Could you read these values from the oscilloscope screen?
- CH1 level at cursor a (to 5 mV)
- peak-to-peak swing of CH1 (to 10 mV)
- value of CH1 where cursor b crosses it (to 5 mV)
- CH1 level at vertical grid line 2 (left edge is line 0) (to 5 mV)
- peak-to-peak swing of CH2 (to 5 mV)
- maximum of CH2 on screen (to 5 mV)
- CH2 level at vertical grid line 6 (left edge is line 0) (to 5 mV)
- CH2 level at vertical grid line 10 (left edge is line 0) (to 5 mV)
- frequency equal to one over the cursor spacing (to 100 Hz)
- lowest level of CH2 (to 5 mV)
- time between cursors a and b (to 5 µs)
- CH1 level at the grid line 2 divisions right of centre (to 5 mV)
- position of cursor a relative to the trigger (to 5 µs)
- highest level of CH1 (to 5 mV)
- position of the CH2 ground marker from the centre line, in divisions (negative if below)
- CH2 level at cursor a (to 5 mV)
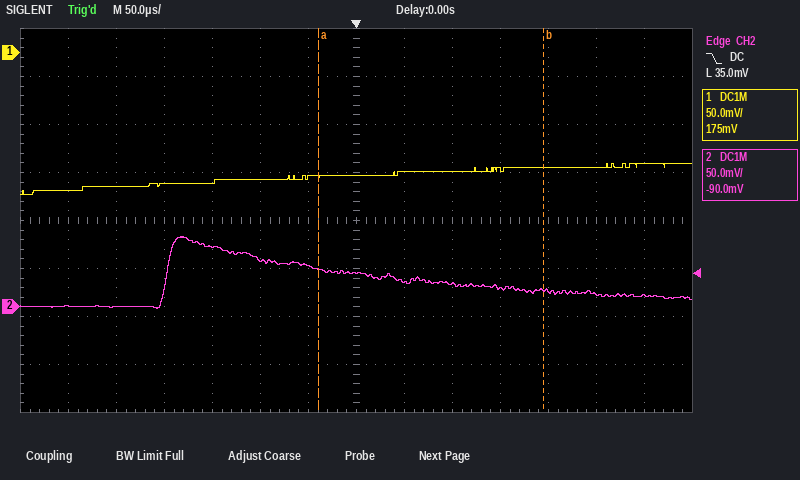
-130 mV
30 mV
-120 mV
-140 mV
75 mV
75 mV
45 mV
20 mV
4.3 kHz
0 mV
235 µs
-125 mV
-40 µs
-115 mV
-1.8 div
40 mV
